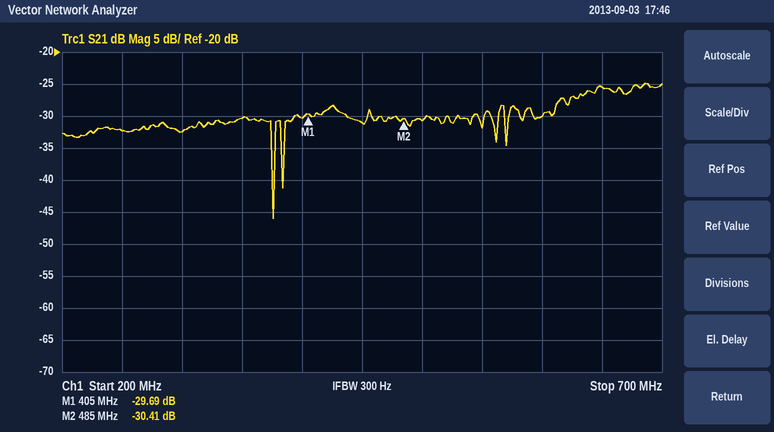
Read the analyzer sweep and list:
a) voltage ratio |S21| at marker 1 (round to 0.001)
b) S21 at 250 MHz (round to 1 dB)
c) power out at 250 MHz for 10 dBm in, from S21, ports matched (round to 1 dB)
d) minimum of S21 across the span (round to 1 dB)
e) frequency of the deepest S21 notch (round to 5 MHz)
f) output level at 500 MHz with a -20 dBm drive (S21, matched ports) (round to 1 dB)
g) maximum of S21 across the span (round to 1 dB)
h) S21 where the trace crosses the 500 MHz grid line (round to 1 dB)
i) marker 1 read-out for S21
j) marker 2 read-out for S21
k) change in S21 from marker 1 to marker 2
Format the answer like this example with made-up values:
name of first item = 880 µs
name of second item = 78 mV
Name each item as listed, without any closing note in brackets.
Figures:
voltage ratio |S21| at marker 1 = 0.033
S21 at 250 MHz = -32 dB
power out at 250 MHz for 10 dBm in, from S21, ports matched = -22 dBm
minimum of S21 across the span = -46 dB
frequency of the deepest S21 notch = 375 MHz
output level at 500 MHz with a -20 dBm drive (S21, matched ports) = -51 dBm
maximum of S21 across the span = -25 dB
S21 where the trace crosses the 500 MHz grid line = -31 dB
marker 1 read-out for S21 = -29.69 dB
marker 2 read-out for S21 = -30.41 dB
change in S21 from marker 1 to marker 2 = -0.72 dB
